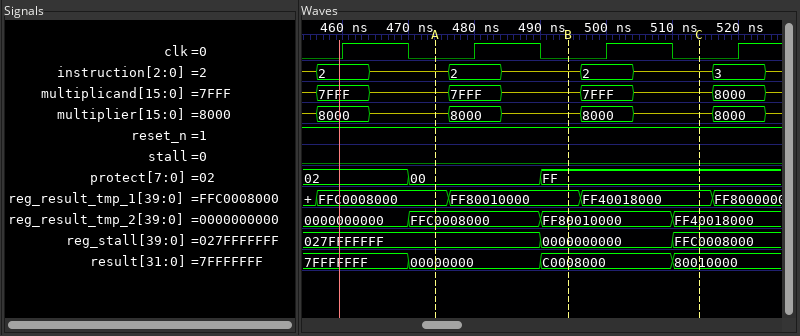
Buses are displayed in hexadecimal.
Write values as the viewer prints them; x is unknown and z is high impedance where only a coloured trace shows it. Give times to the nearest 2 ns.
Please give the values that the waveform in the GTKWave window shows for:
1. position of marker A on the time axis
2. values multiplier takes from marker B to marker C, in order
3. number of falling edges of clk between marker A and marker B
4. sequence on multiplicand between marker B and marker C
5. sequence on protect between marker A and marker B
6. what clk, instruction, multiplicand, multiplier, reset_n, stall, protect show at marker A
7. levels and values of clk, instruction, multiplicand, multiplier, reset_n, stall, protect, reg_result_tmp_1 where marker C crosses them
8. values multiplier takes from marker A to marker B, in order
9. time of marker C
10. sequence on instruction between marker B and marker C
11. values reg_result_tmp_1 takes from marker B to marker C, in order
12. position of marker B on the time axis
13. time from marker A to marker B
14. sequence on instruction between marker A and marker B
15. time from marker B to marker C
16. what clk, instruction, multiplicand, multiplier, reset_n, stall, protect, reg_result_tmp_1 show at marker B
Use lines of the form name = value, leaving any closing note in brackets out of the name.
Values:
position of marker A on the time axis = 474 ns
values multiplier takes from marker B to marker C, in order = z, 8000, z
number of falling edges of clk between marker A and marker B = 1
sequence on multiplicand between marker B and marker C = z, 7FFF, z
sequence on protect between marker A and marker B = 00, FF
what clk, instruction, multiplicand, multiplier, reset_n, stall, protect show at marker A = clk=0, instruction=z, multiplicand=z, multiplier=z, reset_n=1, stall=0, protect=00
levels and values of clk, instruction, multiplicand, multiplier, reset_n, stall, protect, reg_result_tmp_1 where marker C crosses them = clk=0, instruction=z, multiplicand=z, multiplier=z, reset_n=1, stall=0, protect=FF, reg_result_tmp_1=FF40018000
values multiplier takes from marker A to marker B, in order = z, 8000, z
time of marker C = 514 ns
sequence on instruction between marker B and marker C = z, 2, z
values reg_result_tmp_1 takes from marker B to marker C, in order = FF80010000, FF40018000
position of marker B on the time axis = 494 ns
time from marker A to marker B = 20 ns
sequence on instruction between marker A and marker B = z, 2, z
time from marker B to marker C = 20 ns
what clk, instruction, multiplicand, multiplier, reset_n, stall, protect, reg_result_tmp_1 show at marker B = clk=0, instruction=z, multiplicand=z, multiplier=z, reset_n=1, stall=0, protect=FF, reg_result_tmp_1=FF80010000
